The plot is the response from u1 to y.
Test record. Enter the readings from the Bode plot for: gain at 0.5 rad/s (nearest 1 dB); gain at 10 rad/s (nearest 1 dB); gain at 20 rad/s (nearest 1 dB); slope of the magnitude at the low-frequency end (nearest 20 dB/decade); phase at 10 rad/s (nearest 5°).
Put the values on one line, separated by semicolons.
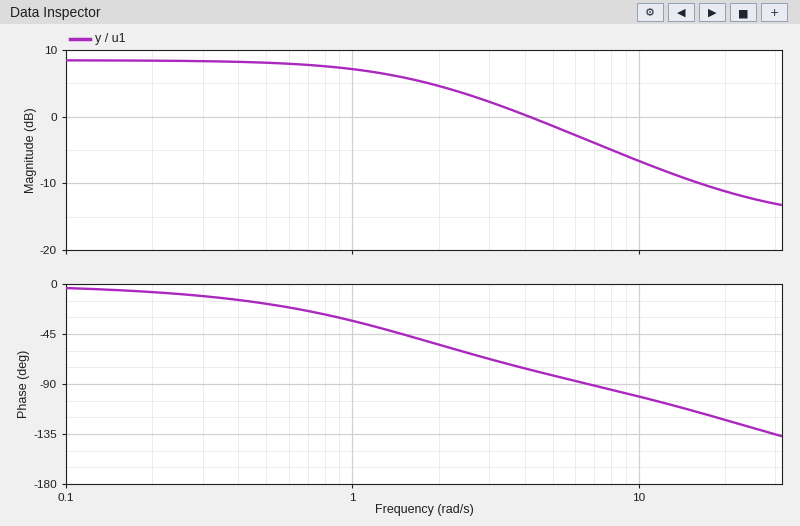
8 dB; -7 dB; -11 dB; 0 dB/decade; -100°
